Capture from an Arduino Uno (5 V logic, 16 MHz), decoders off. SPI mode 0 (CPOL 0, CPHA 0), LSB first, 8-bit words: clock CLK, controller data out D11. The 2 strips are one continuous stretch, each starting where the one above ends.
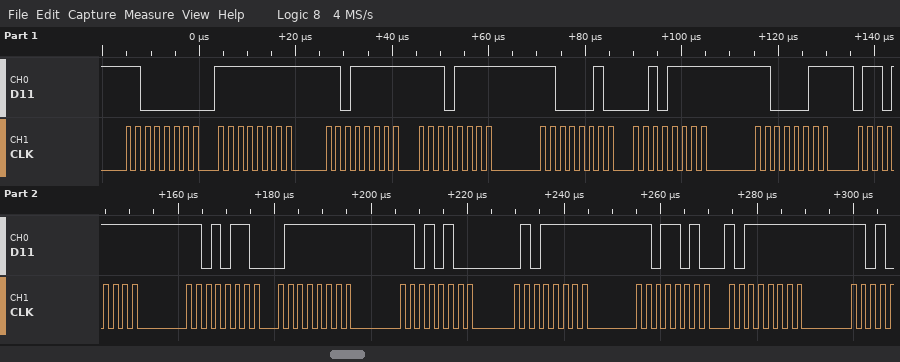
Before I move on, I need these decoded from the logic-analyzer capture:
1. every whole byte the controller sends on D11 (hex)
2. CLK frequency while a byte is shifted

03 FF FB F7 43 F4 C3 F6 6B FE 2B FA 5B FD
500 kHz
